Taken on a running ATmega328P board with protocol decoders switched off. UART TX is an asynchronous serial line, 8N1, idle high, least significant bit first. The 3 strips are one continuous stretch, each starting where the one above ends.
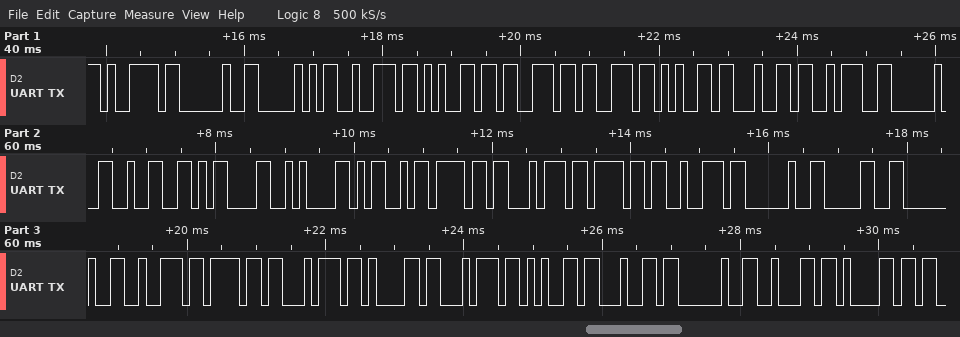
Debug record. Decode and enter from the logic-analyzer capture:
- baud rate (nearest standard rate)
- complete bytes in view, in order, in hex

9600 baud
79 20 50 72 65 73 73 65 64 3A 20 32 0D 0A 4D 6F 74 6F 72 20 30 20 72 6F 74 61 74 65 64 20 62 61
